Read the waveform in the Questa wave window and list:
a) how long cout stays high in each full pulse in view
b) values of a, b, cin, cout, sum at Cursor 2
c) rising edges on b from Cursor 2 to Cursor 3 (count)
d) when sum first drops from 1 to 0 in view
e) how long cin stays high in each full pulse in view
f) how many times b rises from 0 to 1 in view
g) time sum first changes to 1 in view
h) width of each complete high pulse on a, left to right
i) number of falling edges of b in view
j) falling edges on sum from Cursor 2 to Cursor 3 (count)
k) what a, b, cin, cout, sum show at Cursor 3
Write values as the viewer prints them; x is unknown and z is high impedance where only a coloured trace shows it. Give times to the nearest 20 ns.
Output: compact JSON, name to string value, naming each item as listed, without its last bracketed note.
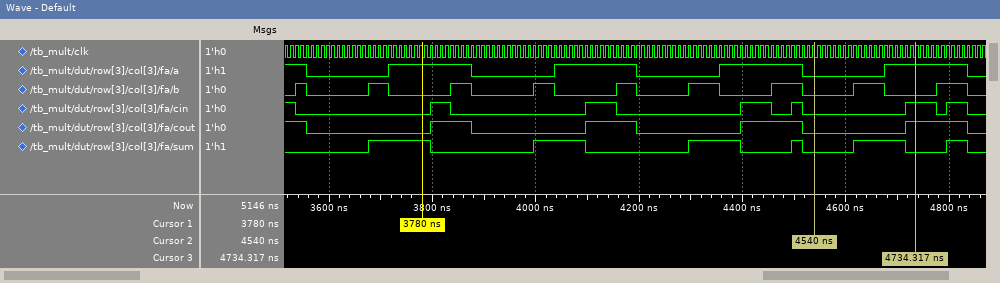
{"how long cout stays high in each full pulse in view": "80 ns, 100 ns, 120 ns, 120 ns", "values of a, b, cin, cout, sum at Cursor 2": "a=0, b=0, cin=0, cout=0, sum=0", "rising edges on b from Cursor 2 to Cursor 3": "1", "when sum first drops from 1 to 0 in view": "3800 ns", "how long cin stays high in each full pulse in view": "40 ns, 60 ns, 60 ns, 20 ns, 60 ns, 40 ns", "how many times b rises from 0 to 1 in view": "9", "time sum first changes to 1 in view": "3680 ns", "width of each complete high pulse on a, left to right": "160 ns, 160 ns, 160 ns, 160 ns", "number of falling edges of b in view": "9", "falling edges on sum from Cursor 2 to Cursor 3": "1", "what a, b, cin, cout, sum show at Cursor 3": "a=1, b=0, cin=1, cout=1, sum=0"}
